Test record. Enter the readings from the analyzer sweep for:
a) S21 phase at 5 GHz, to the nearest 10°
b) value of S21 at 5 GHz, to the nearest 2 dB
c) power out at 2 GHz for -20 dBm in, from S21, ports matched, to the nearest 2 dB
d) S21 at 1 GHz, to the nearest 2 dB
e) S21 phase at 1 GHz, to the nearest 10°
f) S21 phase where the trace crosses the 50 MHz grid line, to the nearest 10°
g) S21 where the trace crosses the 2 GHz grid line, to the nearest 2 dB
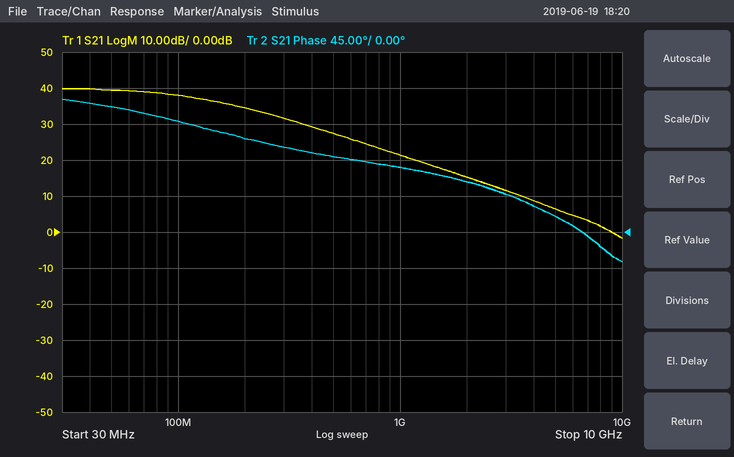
20°
6 dB
-4 dBm
22 dB
80°
160°
16 dB
